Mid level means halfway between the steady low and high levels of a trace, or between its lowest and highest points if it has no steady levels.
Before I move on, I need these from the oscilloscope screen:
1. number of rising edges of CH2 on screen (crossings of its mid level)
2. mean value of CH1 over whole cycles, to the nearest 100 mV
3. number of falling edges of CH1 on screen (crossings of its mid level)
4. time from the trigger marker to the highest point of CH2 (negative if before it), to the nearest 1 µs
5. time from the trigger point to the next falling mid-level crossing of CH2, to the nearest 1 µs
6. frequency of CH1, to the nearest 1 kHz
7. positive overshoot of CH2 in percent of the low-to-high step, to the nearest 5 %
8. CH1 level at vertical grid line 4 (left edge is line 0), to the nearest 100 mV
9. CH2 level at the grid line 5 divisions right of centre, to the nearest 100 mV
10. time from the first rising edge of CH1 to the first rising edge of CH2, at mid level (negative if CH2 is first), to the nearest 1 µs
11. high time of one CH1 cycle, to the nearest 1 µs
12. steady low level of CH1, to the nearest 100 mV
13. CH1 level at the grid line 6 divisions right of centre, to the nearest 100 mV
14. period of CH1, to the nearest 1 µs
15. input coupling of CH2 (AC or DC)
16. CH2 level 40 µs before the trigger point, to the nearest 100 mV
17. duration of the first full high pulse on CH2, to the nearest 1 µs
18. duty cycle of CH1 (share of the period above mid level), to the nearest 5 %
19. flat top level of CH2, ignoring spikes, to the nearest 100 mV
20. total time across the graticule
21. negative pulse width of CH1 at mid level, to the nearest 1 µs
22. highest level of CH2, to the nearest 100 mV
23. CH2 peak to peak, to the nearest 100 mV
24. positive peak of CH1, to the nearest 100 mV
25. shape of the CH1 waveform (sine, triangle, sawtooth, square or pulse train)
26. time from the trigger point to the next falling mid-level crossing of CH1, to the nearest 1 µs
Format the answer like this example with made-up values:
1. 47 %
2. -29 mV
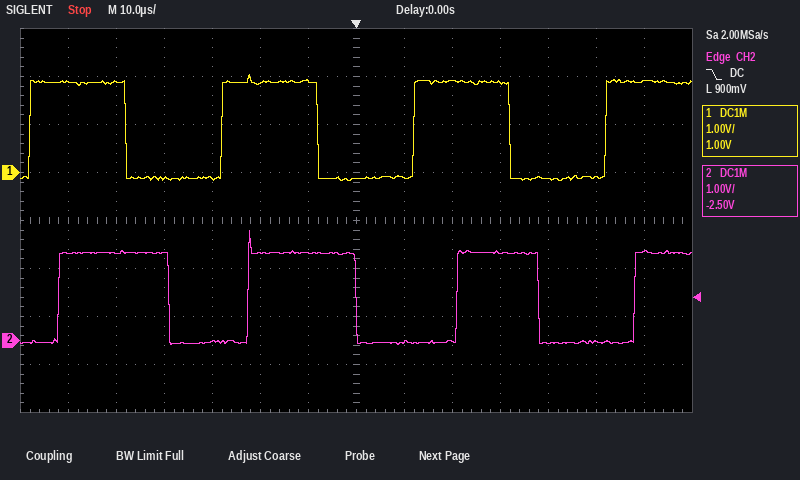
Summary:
1. 4
2. 900 mV
3. 3
4. -22 µs
5. 38 µs
6. 25 kHz
7. 25 %
8. -100 mV
9. 0.0 V
10. +6 µs
11. 20 µs
12. -100 mV
13. 1.9 V
14. 40 µs
15. DC
16. 1.8 V
17. 23 µs
18. 50 %
19. 1.8 V
20. 140 µs
21. 20 µs
22. 2.3 V
23. 2.4 V
24. 2.0 V
25. square
26. 32 µs
